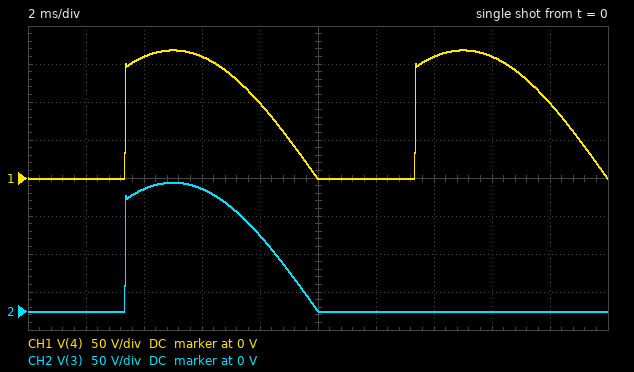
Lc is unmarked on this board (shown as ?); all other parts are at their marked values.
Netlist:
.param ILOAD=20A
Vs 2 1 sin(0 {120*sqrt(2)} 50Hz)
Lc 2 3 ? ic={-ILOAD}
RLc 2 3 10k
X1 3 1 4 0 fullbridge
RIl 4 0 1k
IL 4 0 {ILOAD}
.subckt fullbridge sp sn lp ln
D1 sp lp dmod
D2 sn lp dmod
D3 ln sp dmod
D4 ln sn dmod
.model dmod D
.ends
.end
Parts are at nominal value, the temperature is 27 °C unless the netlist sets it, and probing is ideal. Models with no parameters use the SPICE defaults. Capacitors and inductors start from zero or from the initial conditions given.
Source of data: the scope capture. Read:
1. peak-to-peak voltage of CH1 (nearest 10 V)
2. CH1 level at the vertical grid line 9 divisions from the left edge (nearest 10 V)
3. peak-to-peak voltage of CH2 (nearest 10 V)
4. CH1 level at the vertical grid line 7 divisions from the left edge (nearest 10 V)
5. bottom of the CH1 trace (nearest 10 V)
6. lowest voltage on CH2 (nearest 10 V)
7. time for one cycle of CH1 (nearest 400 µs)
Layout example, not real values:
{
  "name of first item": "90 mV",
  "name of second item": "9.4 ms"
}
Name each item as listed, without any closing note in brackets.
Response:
{
  "peak-to-peak voltage of CH1": "170 V",
  "CH1 level at the vertical grid line 9 divisions from the left edge": "100 V",
  "peak-to-peak voltage of CH2": "170 V",
  "CH1 level at the vertical grid line 7 divisions from the left edge": "160 V",
  "bottom of the CH1 trace": "0 V",
  "lowest voltage on CH2": "0 V",
  "time for one cycle of CH1": "10.0 ms"
}
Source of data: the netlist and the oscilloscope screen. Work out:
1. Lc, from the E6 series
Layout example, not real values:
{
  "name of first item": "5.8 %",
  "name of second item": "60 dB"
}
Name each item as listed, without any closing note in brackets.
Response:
{
  "Lc, from the E6 series": "6.8 mH"
}
